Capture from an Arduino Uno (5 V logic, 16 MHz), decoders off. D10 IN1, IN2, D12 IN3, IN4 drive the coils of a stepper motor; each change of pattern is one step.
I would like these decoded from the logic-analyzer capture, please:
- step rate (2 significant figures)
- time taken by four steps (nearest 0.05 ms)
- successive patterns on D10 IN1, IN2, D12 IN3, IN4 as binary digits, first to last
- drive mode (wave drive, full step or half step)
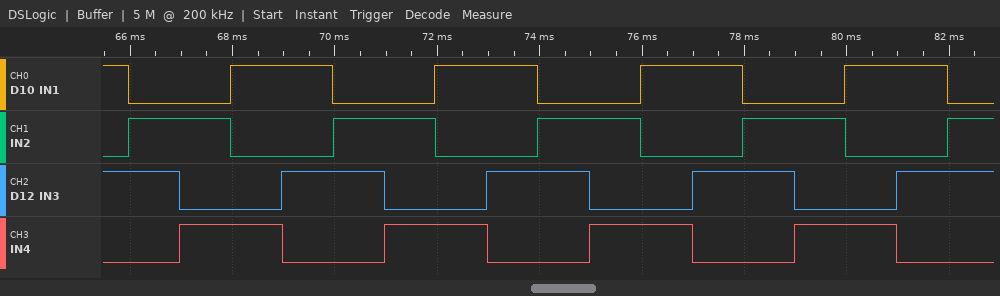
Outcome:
1000 steps/s
4.00 ms
1010 0110 0101 1001 1010 0110 0101 1001 1010 0110 0101 1001 1010 0110 0101 1001 1010 0110
full step
